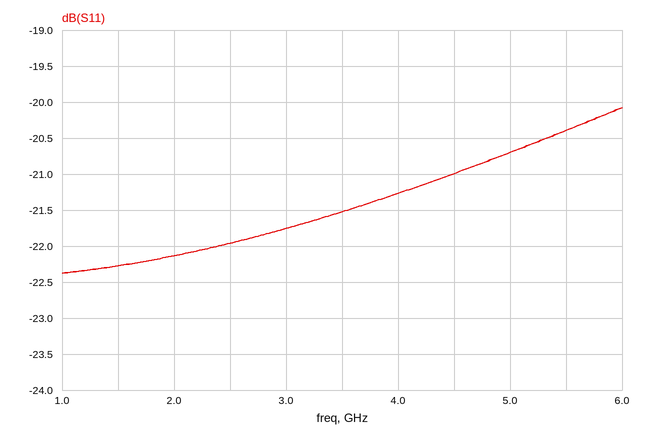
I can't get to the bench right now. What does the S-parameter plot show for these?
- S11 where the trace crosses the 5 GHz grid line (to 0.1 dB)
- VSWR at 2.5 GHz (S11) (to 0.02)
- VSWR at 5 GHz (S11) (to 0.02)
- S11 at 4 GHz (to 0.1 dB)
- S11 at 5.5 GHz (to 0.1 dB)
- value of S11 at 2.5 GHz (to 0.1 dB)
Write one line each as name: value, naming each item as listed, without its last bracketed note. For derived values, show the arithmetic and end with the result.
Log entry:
S11 where the trace crosses the 5 GHz grid line: -20.7 dB
VSWR at 2.5 GHz (S11): |Γ| = 10^(-22/20) = 0.0794; VSWR = (1 + 0.0794)/(1 − 0.0794) ≈ 1.17, so 1.18 to the nearest 0.02
VSWR at 5 GHz (S11): |Γ| = 10^(-20.7/20) = 0.0923; VSWR = (1 + 0.0923)/(1 − 0.0923) ≈ 1.20
S11 at 4 GHz: -21.3 dB
S11 at 5.5 GHz: -20.4 dB
value of S11 at 2.5 GHz: -22.0 dB
